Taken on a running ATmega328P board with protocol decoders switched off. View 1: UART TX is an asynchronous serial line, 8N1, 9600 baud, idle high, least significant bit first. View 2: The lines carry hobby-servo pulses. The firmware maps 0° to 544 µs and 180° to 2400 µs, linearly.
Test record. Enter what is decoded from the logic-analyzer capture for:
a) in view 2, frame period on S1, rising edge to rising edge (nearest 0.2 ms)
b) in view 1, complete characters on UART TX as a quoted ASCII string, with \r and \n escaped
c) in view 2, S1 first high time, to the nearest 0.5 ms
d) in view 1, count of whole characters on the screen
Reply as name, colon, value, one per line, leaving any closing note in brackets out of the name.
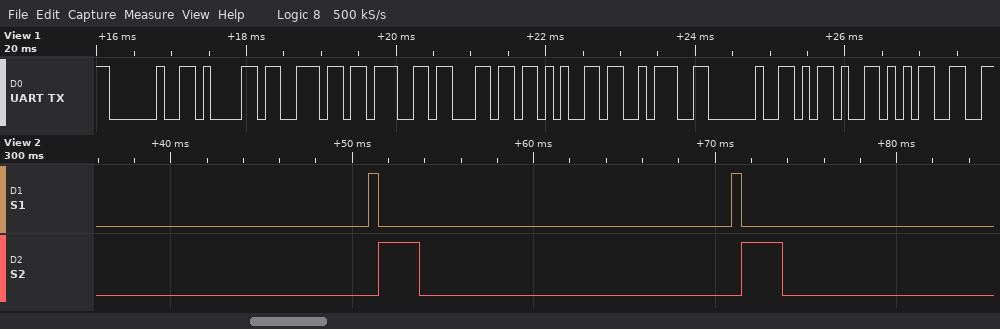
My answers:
in view 2, frame period on S1, rising edge to rising edge: 20.0 ms
in view 1, complete characters on UART TX as a quoted ASCII string, with \r and \n escaped: " angle: -5"
in view 2, S1 first high time, to the nearest 0.5 ms: 0.5 ms
in view 1, count of whole characters on the screen: 10
